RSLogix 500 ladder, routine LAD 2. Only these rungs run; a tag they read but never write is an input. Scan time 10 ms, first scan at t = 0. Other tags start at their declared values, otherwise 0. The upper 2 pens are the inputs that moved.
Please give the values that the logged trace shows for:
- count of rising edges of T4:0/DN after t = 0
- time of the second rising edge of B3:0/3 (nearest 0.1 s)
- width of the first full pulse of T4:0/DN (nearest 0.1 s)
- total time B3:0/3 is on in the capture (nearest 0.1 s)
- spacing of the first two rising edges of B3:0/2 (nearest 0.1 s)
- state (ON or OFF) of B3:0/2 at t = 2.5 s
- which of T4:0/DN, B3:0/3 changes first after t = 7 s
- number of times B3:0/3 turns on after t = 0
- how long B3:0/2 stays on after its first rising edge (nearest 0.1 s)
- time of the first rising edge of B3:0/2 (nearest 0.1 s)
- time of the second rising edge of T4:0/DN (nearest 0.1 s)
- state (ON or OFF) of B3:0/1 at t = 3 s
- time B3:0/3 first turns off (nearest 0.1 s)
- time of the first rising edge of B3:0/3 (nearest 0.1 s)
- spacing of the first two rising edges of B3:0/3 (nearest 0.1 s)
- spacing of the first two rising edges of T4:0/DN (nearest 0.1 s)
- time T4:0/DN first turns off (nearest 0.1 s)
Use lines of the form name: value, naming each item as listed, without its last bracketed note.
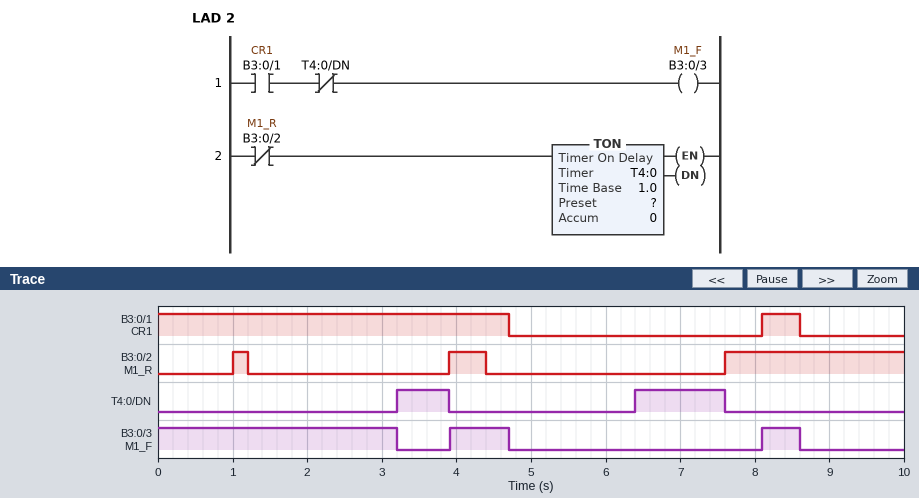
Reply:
count of rising edges of T4:0/DN after t = 0: 2
time of the second rising edge of B3:0/3: 8.1 s
width of the first full pulse of T4:0/DN: 0.7 s
total time B3:0/3 is on in the capture: 4.5 s
spacing of the first two rising edges of B3:0/2: 2.9 s
state (ON or OFF) of B3:0/2 at t = 2.5 s: OFF
which of T4:0/DN, B3:0/3 changes first after t = 7 s: T4:0/DN
number of times B3:0/3 turns on after t = 0: 2
how long B3:0/2 stays on after its first rising edge: 0.2 s
time of the first rising edge of B3:0/2: 1.0 s
time of the second rising edge of T4:0/DN: 6.4 s
state (ON or OFF) of B3:0/1 at t = 3 s: ON
time B3:0/3 first turns off: 3.2 s
time of the first rising edge of B3:0/3: 3.9 s
spacing of the first two rising edges of B3:0/3: 4.2 s
spacing of the first two rising edges of T4:0/DN: 3.2 s
time T4:0/DN first turns off: 3.9 s
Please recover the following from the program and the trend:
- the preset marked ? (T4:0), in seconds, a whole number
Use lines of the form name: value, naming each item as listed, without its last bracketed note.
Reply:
the preset marked ? (T4:0), in seconds, a whole number: 2 s
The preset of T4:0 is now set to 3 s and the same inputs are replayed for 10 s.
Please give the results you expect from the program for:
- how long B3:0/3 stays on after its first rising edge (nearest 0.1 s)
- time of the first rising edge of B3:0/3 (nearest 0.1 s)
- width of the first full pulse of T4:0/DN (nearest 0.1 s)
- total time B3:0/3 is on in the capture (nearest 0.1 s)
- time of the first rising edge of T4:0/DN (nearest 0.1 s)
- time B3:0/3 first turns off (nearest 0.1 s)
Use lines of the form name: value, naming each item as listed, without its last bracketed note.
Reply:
how long B3:0/3 stays on after its first rising edge: 0.5 s
time of the first rising edge of B3:0/3: 8.1 s
width of the first full pulse of T4:0/DN: 0.2 s
total time B3:0/3 is on in the capture: 5.2 s
time of the first rising edge of T4:0/DN: 7.4 s
time B3:0/3 first turns off: 4.7 s
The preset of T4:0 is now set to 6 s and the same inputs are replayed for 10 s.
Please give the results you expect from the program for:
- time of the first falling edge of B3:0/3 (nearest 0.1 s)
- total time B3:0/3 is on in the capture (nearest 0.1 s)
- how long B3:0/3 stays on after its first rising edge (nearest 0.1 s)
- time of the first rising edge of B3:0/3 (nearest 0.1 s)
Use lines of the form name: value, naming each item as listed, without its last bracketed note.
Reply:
time of the first falling edge of B3:0/3: 4.7 s
total time B3:0/3 is on in the capture: 5.2 s
how long B3:0/3 stays on after its first rising edge: 0.5 s
time of the first rising edge of B3:0/3: 8.1 s
